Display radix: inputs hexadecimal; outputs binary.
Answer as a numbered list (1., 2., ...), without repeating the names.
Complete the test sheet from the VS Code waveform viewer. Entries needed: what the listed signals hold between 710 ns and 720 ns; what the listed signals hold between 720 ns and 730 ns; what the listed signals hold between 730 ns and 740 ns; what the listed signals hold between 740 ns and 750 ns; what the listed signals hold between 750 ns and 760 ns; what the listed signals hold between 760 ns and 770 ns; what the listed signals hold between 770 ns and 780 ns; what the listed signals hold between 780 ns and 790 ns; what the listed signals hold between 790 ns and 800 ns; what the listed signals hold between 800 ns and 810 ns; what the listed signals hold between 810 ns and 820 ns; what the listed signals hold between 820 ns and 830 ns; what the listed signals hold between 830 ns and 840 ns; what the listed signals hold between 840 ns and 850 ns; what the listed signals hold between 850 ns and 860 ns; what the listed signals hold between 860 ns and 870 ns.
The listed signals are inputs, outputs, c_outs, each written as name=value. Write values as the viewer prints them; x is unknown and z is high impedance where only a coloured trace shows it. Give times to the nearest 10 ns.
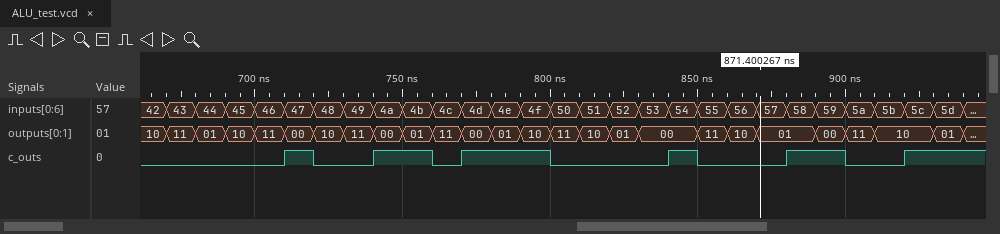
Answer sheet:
1. inputs=47, outputs=00, c_outs=1
2. inputs=48, outputs=10, c_outs=0
3. inputs=49, outputs=11, c_outs=0
4. inputs=4a, outputs=00, c_outs=1
5. inputs=4b, outputs=01, c_outs=1
6. inputs=4c, outputs=11, c_outs=0
7. inputs=4d, outputs=00, c_outs=1
8. inputs=4e, outputs=01, c_outs=1
9. inputs=4f, outputs=10, c_outs=1
10. inputs=50, outputs=11, c_outs=0
11. inputs=51, outputs=10, c_outs=0
12. inputs=52, outputs=01, c_outs=0
13. inputs=53, outputs=00, c_outs=0
14. inputs=54, outputs=00, c_outs=1
15. inputs=55, outputs=11, c_outs=0
16. inputs=56, outputs=10, c_outs=0
